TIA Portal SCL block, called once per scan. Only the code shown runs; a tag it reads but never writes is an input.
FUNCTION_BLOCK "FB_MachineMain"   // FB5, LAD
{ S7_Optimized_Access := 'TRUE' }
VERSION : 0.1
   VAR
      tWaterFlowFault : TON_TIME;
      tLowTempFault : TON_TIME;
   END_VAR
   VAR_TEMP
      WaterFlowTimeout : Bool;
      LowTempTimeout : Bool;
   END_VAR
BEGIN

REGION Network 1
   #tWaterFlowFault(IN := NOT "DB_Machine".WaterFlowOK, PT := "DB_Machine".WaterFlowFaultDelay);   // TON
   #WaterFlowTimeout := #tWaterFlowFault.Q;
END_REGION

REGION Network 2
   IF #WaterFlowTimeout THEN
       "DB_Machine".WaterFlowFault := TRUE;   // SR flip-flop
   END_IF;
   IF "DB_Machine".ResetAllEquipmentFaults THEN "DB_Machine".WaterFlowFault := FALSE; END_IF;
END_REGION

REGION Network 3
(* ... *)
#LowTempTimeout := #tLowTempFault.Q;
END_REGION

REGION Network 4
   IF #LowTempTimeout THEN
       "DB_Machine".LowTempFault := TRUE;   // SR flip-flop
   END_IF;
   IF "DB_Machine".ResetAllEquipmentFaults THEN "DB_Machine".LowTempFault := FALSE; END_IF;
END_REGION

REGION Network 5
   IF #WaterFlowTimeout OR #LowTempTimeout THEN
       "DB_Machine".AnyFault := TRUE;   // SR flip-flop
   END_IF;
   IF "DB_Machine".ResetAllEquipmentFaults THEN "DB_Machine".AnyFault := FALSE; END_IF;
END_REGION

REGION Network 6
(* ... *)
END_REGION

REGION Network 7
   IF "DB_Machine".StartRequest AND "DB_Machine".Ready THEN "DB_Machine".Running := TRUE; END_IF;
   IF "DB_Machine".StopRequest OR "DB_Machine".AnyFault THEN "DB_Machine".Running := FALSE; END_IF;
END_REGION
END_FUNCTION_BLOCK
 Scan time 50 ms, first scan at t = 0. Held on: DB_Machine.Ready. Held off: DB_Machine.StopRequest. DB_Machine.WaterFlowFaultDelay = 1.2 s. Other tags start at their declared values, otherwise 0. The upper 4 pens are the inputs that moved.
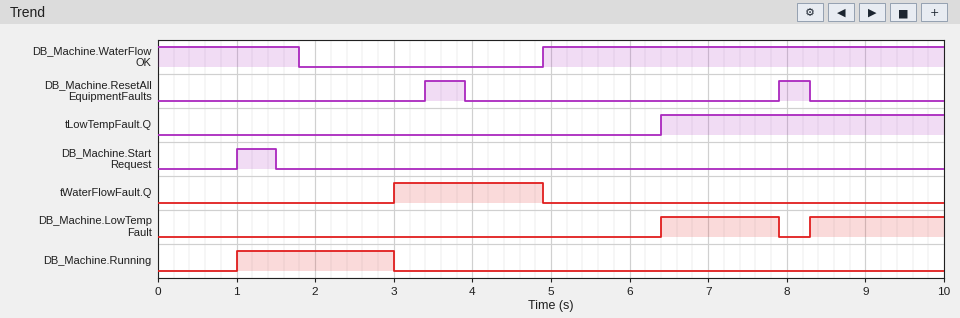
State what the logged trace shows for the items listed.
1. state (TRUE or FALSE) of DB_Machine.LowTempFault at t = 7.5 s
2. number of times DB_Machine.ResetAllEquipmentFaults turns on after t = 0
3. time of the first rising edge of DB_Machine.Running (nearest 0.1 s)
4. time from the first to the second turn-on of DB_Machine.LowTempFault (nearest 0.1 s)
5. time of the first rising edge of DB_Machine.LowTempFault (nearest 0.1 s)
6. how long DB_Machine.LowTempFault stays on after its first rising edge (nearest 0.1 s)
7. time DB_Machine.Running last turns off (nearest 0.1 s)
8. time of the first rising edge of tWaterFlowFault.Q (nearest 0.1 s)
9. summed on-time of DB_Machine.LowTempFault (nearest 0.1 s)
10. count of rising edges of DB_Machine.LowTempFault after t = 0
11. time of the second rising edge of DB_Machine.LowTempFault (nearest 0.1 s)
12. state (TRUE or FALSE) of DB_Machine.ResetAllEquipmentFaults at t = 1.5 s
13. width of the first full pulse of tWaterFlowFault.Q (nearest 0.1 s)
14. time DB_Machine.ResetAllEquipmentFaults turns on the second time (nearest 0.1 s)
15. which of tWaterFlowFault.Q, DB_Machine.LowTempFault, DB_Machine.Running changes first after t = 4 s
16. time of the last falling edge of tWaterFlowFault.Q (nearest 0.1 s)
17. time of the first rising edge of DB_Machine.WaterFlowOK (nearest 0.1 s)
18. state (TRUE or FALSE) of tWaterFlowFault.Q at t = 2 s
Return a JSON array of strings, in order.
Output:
["TRUE", "2", "1.0 s", "1.9 s", "6.4 s", "1.5 s", "3.0 s", "3.0 s", "3.2 s", "2", "8.3 s", "FALSE", "1.9 s", "7.9 s", "tWaterFlowFault.Q", "4.9 s", "4.9 s", "FALSE"]
